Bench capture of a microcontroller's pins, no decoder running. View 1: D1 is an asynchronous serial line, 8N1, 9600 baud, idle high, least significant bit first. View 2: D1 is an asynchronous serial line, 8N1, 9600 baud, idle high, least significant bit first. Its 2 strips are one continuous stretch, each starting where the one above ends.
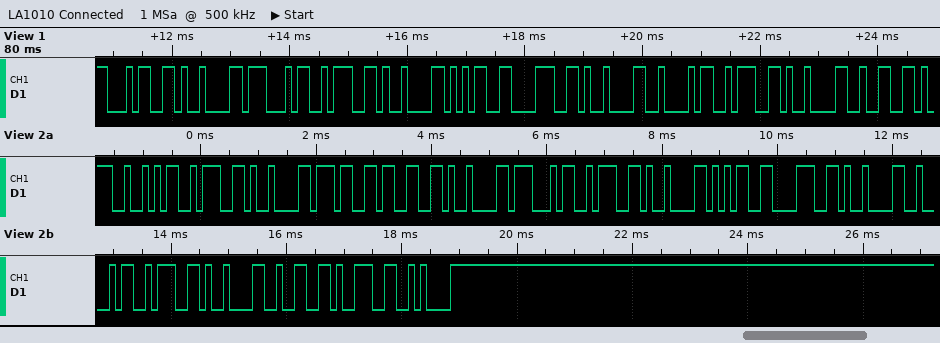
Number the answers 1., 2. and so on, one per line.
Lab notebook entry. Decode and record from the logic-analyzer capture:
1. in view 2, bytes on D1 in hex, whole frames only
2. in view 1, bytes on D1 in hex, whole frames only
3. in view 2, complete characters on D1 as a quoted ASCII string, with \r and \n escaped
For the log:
1. 0x52 0x3A 0x09 0x37 0x33 0x09 0x47 0x3A 0x09 0x35 0x38 0x09 0x42 0x3A 0x09 0x32 0x39 0x0A
2. 34 09 47 3A 09 35 38 09 42 3A 09 32
3. "R:\t73\tG:\t58\tB:\t29\n"
